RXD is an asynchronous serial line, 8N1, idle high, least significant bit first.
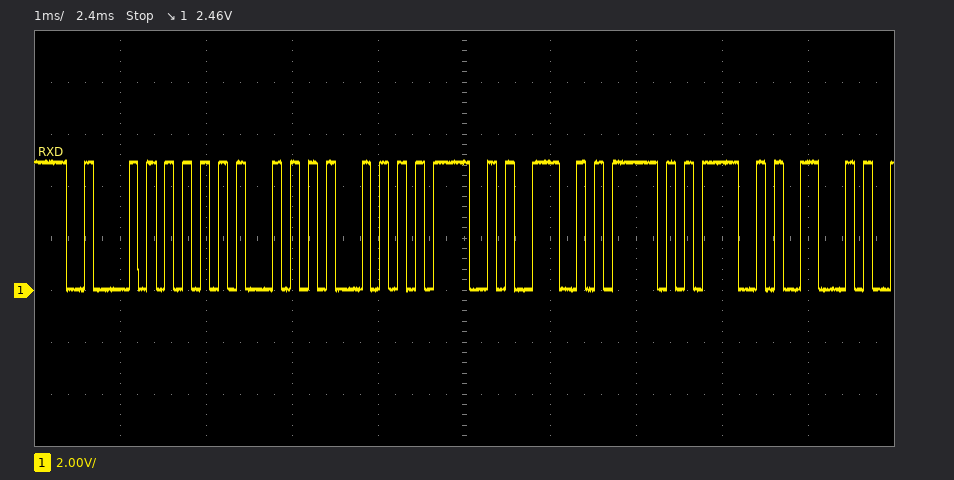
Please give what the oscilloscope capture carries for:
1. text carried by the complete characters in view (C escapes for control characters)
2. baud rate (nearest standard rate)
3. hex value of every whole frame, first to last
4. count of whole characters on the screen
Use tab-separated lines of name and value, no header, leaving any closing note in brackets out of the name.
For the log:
text carried by the complete characters in view	"BUTTON_OF"
baud rate	9600 baud
hex value of every whole frame, first to last	0x42 0x55 0x54 0x54 0x4F 0x4E 0x5F 0x4F 0x46
count of whole characters on the screen	9
